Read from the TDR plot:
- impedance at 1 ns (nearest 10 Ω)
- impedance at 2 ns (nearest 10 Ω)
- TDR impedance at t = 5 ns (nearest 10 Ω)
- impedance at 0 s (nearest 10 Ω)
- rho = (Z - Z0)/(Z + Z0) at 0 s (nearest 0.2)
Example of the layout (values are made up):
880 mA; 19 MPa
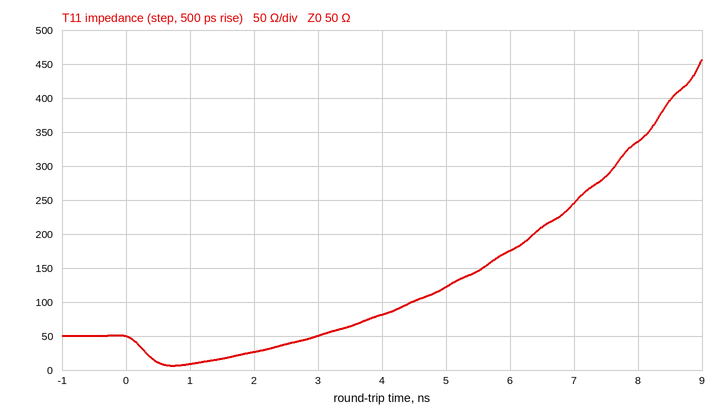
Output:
10 Ω; 30 Ω; 120 Ω; 50 Ω; 0.0
